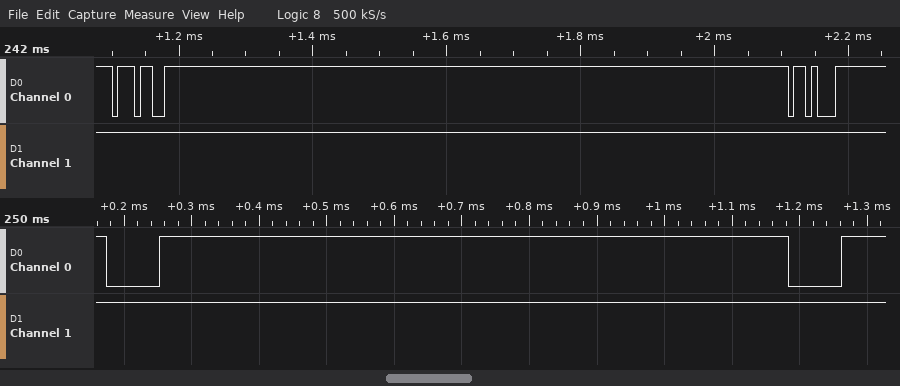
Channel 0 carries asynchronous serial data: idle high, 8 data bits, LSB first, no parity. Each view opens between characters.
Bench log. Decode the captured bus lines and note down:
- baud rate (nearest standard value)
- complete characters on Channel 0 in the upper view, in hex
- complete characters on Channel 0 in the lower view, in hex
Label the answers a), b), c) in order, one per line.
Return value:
a) 115200 baud
b) 37, 8B
c) 00, 00
